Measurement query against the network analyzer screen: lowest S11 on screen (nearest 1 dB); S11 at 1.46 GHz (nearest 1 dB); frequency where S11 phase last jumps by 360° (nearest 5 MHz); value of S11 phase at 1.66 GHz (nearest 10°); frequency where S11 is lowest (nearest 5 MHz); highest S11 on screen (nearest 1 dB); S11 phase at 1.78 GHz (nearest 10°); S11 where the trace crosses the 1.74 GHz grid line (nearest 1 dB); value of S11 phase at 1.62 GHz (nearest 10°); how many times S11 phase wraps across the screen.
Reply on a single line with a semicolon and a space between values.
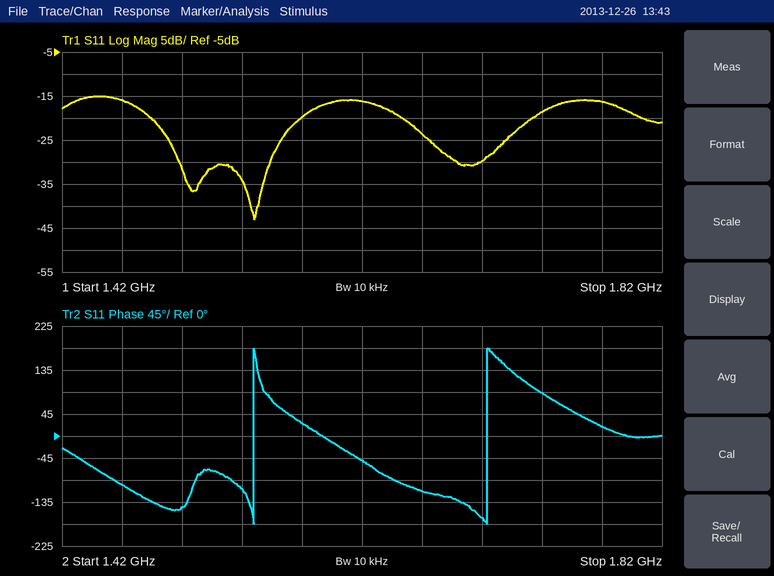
-43 dB; -16 dB; 1.705 GHz; -110°; 1.550 GHz; -15 dB; 20°; -19 dB; -50°; 2
